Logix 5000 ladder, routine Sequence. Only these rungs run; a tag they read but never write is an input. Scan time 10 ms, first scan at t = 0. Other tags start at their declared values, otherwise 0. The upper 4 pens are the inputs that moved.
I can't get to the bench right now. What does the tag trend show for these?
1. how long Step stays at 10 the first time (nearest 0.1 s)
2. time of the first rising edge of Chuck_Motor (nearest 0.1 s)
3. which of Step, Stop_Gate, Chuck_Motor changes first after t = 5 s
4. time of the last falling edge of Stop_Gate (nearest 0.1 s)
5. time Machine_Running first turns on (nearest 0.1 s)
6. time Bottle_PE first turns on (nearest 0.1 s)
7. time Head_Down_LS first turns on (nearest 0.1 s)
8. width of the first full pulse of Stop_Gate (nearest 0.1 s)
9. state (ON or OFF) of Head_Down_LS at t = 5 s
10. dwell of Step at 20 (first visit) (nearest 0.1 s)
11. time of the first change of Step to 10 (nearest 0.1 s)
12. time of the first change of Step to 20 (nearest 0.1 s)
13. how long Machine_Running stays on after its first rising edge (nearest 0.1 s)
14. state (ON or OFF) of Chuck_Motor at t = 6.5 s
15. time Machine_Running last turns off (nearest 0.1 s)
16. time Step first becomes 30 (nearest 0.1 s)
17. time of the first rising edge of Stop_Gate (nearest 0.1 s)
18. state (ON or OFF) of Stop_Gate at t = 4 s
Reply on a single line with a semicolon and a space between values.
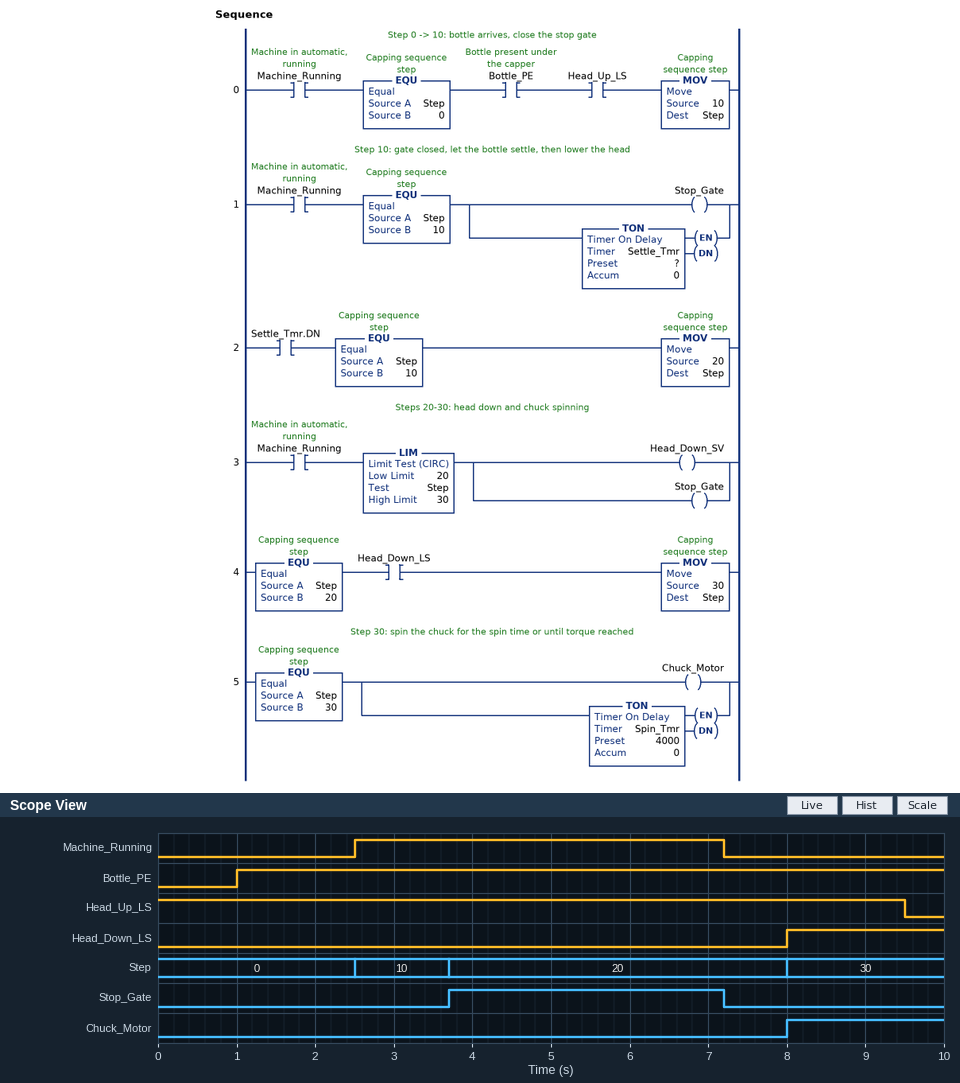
1.2 s; 8.0 s; Stop_Gate; 7.2 s; 2.5 s; 1.0 s; 8.0 s; 3.5 s; OFF; 4.3 s; 2.5 s; 3.7 s; 4.7 s; OFF; 7.2 s; 8.0 s; 3.7 s; ON
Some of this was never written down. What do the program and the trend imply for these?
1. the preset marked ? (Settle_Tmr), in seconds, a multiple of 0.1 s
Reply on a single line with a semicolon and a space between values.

1.2 s
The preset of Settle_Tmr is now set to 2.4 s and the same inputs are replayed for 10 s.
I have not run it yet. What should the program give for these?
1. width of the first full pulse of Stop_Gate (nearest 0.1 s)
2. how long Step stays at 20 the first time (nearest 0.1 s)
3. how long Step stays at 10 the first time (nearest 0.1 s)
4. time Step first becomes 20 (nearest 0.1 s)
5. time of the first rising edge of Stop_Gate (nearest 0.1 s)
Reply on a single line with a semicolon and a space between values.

2.3 s; 3.1 s; 2.4 s; 4.9 s; 4.9 s
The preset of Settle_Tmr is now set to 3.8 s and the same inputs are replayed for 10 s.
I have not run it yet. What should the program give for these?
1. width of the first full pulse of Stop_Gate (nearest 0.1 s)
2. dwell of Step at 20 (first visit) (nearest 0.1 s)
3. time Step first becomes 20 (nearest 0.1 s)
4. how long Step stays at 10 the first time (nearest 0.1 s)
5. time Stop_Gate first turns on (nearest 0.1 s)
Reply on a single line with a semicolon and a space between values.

0.9 s; 1.7 s; 6.3 s; 3.8 s; 6.3 s
